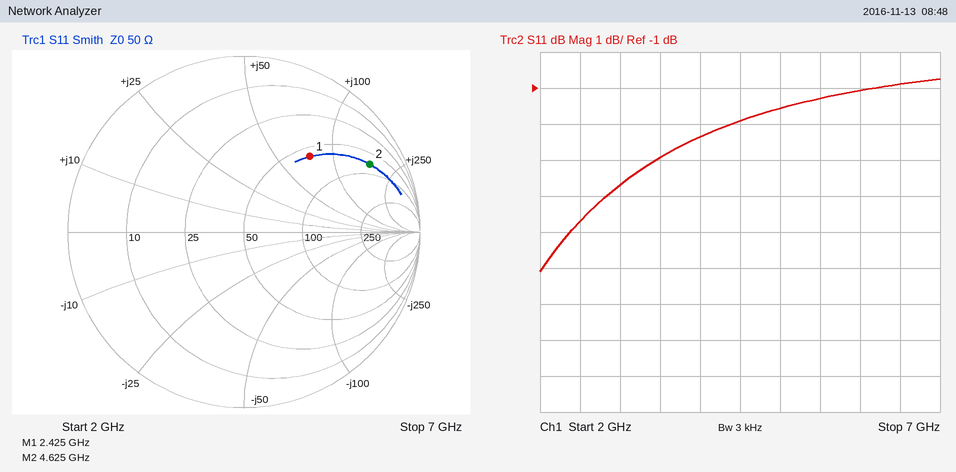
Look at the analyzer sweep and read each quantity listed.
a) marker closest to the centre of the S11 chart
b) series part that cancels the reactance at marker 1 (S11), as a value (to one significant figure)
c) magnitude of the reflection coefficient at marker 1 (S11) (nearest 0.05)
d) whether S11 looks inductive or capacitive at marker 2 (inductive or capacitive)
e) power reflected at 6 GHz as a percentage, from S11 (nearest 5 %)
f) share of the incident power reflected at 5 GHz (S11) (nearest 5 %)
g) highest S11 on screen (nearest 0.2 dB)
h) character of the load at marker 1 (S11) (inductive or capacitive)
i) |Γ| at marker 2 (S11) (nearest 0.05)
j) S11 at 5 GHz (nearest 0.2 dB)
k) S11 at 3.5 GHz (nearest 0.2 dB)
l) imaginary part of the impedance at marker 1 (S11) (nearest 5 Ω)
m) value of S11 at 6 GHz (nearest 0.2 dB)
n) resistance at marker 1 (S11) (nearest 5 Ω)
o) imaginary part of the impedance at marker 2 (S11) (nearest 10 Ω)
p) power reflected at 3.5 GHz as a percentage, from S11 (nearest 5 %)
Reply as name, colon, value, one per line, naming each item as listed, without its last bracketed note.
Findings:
marker closest to the centre of the S11 chart: marker 1
series part that cancels the reactance at marker 1 (S11), as a value: 900 fF
magnitude of the reflection coefficient at marker 1 (S11): 0.55
whether S11 looks inductive or capacitive at marker 2: inductive
power reflected at 6 GHz as a percentage, from S11: 80 %
share of the incident power reflected at 5 GHz (S11): 70 %
highest S11 on screen: -0.8 dB
character of the load at marker 1 (S11): inductive
|Γ| at marker 2 (S11): 0.80
S11 at 5 GHz: -1.6 dB
S11 at 3.5 GHz: -3.0 dB
imaginary part of the impedance at marker 1 (S11): +75 Ω
value of S11 at 6 GHz: -1.0 dB
resistance at marker 1 (S11): 60 Ω
imaginary part of the impedance at marker 2 (S11): +170 Ω
power reflected at 3.5 GHz as a percentage, from S11: 50 %
